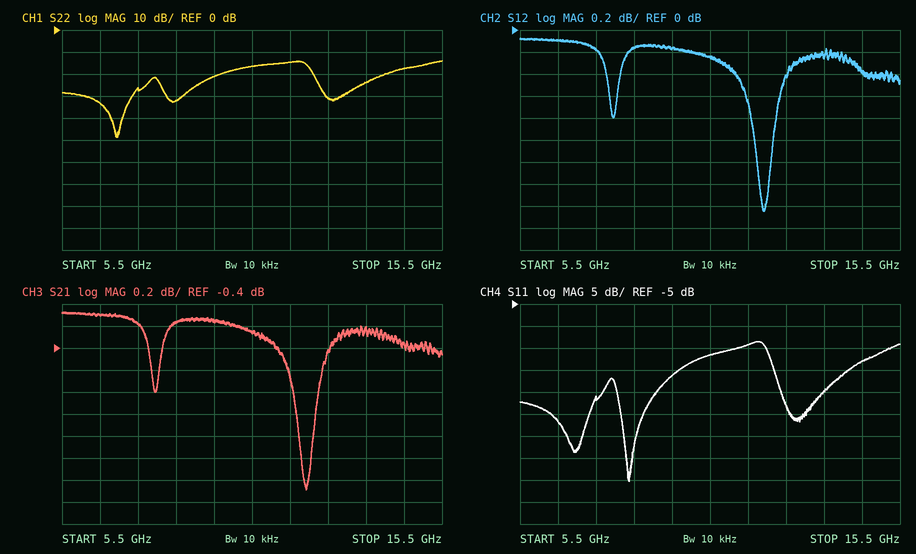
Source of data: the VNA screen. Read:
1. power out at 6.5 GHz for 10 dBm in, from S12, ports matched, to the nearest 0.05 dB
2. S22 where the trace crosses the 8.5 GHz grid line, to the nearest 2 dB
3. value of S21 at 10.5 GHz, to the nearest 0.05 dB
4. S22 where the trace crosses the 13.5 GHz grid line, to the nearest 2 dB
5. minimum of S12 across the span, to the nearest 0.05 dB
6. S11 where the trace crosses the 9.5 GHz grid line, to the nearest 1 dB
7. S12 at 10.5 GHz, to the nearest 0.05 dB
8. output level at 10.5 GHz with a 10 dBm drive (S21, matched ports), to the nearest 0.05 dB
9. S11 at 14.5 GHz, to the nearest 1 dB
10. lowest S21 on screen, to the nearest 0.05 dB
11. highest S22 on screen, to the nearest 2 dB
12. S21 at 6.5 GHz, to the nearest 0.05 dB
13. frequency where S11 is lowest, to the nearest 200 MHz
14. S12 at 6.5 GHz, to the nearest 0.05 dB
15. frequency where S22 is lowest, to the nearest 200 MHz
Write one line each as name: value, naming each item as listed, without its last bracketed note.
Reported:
power out at 6.5 GHz for 10 dBm in, from S12, ports matched, to the nearest 0.05 dB: 9.90 dBm
S22 where the trace crosses the 8.5 GHz grid line, to the nearest 2 dB: -32 dB
value of S21 at 10.5 GHz, to the nearest 0.05 dB: -0.25 dB
S22 where the trace crosses the 13.5 GHz grid line, to the nearest 2 dB: -24 dB
minimum of S12 across the span, to the nearest 0.05 dB: -1.65 dB
S11 where the trace crosses the 9.5 GHz grid line, to the nearest 1 dB: -21 dB
S12 at 10.5 GHz, to the nearest 0.05 dB: -0.25 dB
output level at 10.5 GHz with a 10 dBm drive (S21, matched ports), to the nearest 0.05 dB: 9.75 dBm
S11 at 14.5 GHz, to the nearest 1 dB: -18 dB
lowest S21 on screen, to the nearest 0.05 dB: -1.70 dB
highest S22 on screen, to the nearest 2 dB: -14 dB
S21 at 6.5 GHz, to the nearest 0.05 dB: -0.10 dB
frequency where S11 is lowest, to the nearest 200 MHz: 8.4 GHz
S12 at 6.5 GHz, to the nearest 0.05 dB: -0.10 dB
frequency where S22 is lowest, to the nearest 200 MHz: 7.0 GHz
